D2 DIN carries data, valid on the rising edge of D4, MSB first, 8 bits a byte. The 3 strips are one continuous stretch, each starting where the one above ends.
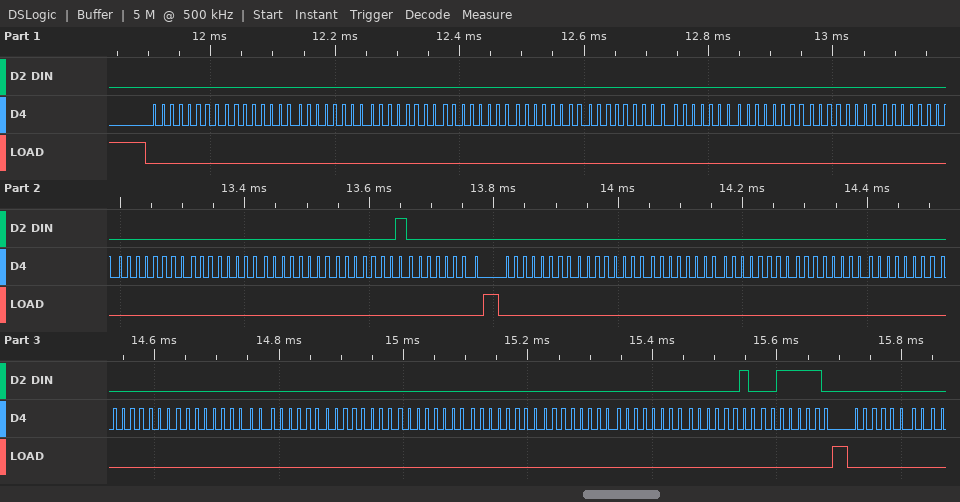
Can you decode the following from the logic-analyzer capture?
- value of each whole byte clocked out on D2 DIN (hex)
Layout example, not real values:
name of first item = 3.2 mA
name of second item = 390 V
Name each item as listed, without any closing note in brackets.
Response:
value of each whole byte clocked out on D2 DIN = 00 00 00 00 00 00 00 00 00 00 00 00 00 00 01 00 00 00 00 00 00 00 00 00 00 00 00 00 00 00 02 3E 00
